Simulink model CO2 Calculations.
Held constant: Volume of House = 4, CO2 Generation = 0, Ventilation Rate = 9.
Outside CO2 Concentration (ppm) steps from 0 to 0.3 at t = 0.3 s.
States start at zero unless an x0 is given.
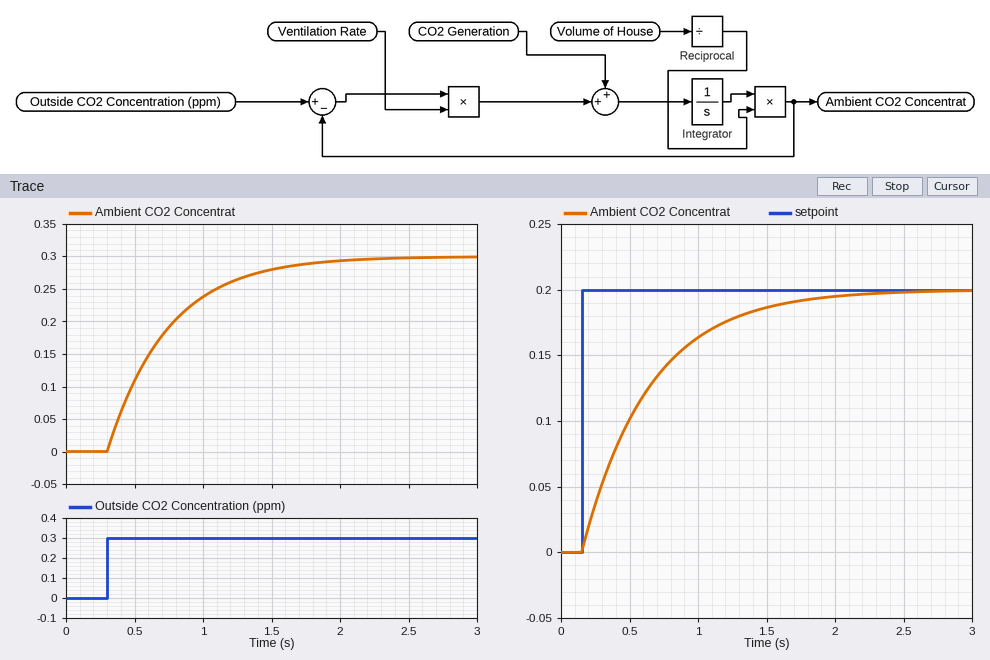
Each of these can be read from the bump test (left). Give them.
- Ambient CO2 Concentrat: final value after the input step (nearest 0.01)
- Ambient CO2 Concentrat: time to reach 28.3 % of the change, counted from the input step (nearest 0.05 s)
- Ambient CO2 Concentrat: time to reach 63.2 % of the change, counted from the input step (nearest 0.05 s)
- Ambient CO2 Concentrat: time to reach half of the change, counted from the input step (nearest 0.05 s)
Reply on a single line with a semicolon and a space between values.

0.30; 0.15 s; 0.45 s; 0.30 s
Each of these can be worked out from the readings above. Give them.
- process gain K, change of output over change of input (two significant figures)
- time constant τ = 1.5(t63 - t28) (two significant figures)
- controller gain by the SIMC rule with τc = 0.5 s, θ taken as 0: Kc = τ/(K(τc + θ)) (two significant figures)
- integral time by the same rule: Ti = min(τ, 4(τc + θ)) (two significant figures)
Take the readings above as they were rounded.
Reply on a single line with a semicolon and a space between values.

1.0; 0.45 s; 0.90; 0.45 s
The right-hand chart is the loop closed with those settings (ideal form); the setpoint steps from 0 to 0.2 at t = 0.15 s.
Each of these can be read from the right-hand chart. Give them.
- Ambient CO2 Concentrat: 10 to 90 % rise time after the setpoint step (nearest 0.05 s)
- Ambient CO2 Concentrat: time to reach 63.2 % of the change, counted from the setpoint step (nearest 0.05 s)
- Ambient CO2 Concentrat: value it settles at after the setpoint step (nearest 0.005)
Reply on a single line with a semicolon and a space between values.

1.10 s; 0.50 s; 0.200
